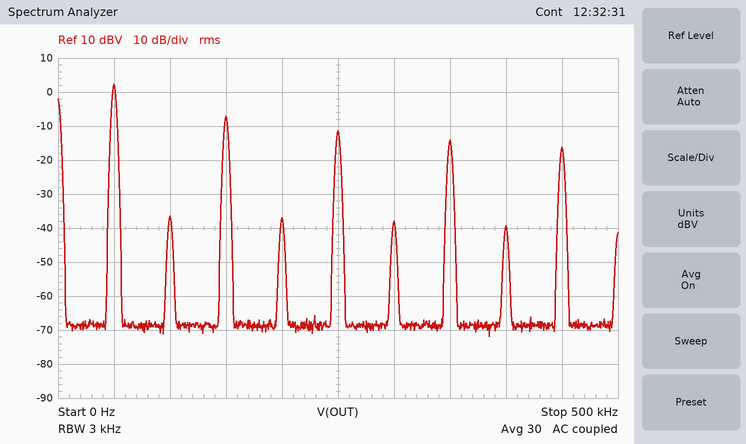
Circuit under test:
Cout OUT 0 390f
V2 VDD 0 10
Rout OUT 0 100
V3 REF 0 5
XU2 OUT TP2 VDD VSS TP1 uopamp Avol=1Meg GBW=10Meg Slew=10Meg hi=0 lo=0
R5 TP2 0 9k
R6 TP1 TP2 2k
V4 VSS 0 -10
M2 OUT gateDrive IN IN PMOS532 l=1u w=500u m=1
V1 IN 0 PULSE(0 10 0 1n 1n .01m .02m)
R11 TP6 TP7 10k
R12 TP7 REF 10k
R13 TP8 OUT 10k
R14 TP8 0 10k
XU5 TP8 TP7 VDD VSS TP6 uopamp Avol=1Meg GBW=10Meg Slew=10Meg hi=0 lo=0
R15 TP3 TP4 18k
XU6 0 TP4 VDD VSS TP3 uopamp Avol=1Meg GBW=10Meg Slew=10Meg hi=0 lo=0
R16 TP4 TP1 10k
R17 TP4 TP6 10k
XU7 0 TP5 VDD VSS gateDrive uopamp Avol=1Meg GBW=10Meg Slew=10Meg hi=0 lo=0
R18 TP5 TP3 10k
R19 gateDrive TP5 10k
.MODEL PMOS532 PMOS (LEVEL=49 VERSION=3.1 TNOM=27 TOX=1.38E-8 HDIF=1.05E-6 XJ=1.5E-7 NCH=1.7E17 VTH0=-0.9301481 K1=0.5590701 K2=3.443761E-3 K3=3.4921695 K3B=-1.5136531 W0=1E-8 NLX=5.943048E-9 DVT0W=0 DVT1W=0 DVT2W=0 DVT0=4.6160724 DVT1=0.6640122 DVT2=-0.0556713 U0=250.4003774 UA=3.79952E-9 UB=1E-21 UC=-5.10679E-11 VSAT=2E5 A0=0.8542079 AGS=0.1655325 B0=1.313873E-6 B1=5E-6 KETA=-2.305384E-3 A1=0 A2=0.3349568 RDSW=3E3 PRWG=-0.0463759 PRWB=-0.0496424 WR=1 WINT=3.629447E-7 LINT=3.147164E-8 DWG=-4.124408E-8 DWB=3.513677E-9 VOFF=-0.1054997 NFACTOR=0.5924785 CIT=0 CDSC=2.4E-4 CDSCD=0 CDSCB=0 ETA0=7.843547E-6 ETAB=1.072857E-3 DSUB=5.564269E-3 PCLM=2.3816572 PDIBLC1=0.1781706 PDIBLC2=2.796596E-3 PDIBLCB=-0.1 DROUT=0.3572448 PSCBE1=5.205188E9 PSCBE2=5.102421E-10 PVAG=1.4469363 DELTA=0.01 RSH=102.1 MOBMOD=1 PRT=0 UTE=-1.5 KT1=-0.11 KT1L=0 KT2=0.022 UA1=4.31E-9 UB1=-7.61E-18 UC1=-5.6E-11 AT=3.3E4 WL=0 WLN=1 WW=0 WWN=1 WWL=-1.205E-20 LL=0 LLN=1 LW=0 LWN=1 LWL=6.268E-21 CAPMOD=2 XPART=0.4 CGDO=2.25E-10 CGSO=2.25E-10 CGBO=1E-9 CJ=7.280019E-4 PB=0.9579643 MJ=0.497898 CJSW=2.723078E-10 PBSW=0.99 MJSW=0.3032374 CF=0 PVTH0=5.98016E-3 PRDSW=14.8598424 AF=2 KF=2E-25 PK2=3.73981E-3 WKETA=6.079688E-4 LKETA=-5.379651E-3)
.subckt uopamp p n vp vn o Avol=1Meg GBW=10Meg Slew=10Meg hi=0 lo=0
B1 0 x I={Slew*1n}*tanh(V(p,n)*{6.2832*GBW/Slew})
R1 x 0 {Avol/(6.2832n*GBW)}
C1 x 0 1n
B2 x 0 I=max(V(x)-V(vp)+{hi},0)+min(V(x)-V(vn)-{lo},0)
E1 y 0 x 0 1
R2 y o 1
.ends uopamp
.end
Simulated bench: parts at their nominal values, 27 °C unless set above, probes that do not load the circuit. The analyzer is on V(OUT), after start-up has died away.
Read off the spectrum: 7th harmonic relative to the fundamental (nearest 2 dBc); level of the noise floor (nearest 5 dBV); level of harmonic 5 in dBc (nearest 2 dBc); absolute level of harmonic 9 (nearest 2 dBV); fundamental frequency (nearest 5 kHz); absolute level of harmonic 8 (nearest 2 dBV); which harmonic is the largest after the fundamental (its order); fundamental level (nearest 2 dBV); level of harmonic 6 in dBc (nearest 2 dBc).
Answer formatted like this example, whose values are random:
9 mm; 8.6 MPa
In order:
-16 dBc; -70 dBV; -14 dBc; -16 dBV; 50 kHz; -40 dBV; 3; 2 dBV; -40 dBc
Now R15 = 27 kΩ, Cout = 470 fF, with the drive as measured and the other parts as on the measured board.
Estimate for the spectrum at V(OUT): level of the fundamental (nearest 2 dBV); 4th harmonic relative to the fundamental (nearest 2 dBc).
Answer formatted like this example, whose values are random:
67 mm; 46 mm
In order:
2 dBV; -34 dBc
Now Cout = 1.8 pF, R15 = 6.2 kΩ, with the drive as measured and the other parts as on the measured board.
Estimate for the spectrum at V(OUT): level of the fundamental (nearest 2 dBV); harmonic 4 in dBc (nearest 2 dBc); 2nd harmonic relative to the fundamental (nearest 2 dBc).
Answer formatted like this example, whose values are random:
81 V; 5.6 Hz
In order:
2 dBV; -56 dBc; -56 dBc
